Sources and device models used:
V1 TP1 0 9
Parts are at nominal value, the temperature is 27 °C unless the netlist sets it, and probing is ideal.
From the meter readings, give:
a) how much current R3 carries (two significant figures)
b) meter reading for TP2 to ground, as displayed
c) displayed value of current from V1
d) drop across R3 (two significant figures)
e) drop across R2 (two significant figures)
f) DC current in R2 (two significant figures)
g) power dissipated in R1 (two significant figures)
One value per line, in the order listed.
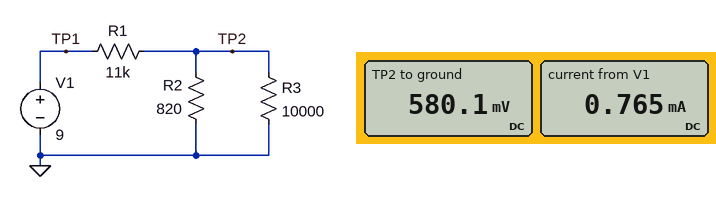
58 µA
580.1 mV
0.765 mA
580 mV
580 mV
710 µA
6.4 mW
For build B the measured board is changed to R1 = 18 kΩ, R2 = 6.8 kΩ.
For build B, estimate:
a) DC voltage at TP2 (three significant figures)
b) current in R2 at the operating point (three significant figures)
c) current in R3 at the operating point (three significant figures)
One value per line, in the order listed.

1.65 V
243 µA
165 µA
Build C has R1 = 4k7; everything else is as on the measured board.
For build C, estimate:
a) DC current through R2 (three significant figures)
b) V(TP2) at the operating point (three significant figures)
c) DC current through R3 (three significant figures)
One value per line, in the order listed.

1.52 mA
1.25 V
125 µA
